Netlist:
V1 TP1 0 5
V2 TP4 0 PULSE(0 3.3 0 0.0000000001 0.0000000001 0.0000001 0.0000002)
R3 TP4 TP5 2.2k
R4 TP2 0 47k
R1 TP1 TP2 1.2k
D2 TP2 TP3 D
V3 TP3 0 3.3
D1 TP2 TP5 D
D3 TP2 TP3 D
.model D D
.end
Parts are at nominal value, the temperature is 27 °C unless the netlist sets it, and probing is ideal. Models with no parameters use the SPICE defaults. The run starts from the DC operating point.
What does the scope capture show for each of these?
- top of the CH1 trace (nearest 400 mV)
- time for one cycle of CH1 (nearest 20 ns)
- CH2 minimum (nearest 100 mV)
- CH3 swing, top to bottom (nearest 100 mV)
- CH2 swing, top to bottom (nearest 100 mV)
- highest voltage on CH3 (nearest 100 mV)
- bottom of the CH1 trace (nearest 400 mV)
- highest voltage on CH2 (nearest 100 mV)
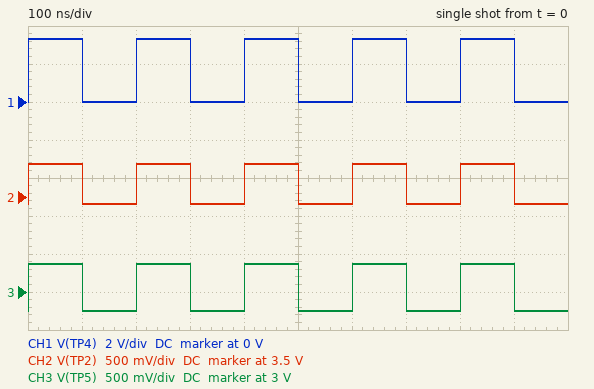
3.2 V
200 ns
3.4 V
600 mV
500 mV
3.4 V
0 V
3.9 V
